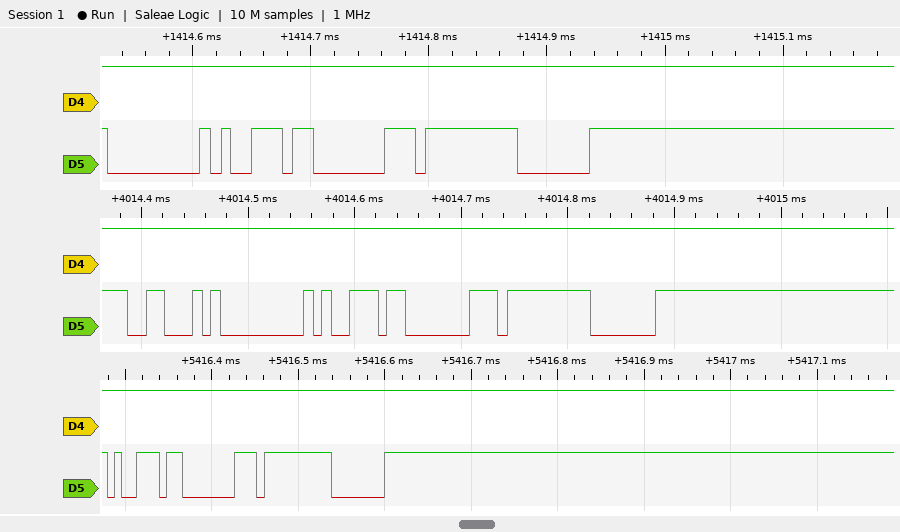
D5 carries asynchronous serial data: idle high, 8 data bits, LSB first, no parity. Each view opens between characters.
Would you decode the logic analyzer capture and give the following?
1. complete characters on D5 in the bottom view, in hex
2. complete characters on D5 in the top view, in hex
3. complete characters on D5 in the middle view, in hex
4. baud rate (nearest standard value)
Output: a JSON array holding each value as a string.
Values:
["B9, C0, FF, C0", "00, B9, C0, FF, C0", "46, 00, B9, C0, FF, C0", "115200 baud"]
